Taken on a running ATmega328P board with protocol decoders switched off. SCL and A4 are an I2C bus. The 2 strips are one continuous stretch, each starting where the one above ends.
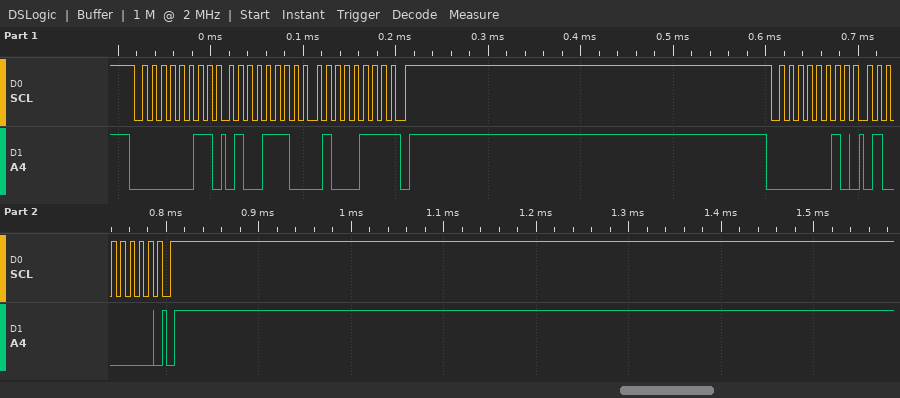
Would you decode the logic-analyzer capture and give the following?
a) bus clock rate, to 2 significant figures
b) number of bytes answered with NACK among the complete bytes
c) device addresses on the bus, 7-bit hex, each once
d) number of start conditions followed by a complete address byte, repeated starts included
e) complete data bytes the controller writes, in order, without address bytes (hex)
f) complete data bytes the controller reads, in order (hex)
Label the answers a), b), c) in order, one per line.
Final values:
a) 100 kHz
b) 1
c) 0x01
d) 2
e) 40
f) 4E 47
